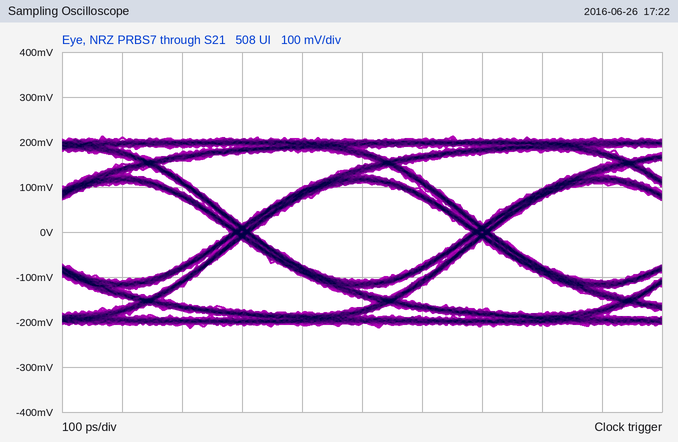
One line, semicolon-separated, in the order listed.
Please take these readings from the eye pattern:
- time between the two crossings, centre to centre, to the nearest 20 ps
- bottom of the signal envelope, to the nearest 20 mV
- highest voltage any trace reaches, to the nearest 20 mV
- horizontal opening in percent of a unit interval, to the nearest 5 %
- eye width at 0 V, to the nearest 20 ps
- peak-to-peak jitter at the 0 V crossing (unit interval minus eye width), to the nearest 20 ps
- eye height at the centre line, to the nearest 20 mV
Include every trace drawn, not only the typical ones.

400 ps; -220 mV; 220 mV; 90 %; 360 ps; 40 ps; 220 mV
